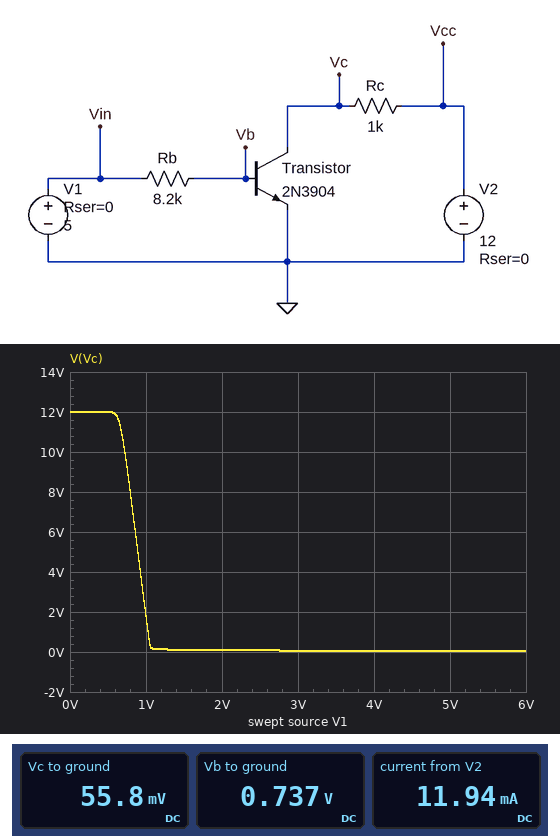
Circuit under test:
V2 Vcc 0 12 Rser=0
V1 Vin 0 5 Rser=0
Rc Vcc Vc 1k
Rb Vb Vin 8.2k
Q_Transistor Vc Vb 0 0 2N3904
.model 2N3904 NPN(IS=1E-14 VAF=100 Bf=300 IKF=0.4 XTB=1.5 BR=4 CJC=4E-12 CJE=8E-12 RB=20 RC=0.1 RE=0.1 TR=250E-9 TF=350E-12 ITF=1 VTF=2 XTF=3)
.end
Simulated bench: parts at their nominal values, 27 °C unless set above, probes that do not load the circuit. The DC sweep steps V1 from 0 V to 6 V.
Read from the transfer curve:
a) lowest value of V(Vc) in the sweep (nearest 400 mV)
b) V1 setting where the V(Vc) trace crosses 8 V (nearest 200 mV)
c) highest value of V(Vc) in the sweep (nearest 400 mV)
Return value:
0 V
800 mV
12.0 V
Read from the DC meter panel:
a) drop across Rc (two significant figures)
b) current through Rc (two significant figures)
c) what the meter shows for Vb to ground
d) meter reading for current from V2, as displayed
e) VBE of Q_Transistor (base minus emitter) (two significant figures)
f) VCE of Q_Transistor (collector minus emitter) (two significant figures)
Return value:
12 V
12 mA
0.737 V
11.94 mA
740 mV
56 mV
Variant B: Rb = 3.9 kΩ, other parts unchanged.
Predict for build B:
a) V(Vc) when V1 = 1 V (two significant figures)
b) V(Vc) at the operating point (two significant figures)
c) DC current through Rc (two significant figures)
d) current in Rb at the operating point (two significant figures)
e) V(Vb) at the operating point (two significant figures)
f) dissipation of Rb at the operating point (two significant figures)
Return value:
120 mV
40 mV
12 mA
1.1 mA
750 mV
4.6 mW
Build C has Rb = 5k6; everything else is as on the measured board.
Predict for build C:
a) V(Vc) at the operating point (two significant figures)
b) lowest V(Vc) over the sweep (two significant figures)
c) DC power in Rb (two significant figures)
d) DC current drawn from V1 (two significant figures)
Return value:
47 mV
43 mV
3.2 mW
760 µA
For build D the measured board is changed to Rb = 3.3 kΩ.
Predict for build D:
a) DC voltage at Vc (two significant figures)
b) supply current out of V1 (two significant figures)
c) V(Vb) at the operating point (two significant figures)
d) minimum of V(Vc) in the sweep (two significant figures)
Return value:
37 mV
1.3 mA
760 mV
34 mV
